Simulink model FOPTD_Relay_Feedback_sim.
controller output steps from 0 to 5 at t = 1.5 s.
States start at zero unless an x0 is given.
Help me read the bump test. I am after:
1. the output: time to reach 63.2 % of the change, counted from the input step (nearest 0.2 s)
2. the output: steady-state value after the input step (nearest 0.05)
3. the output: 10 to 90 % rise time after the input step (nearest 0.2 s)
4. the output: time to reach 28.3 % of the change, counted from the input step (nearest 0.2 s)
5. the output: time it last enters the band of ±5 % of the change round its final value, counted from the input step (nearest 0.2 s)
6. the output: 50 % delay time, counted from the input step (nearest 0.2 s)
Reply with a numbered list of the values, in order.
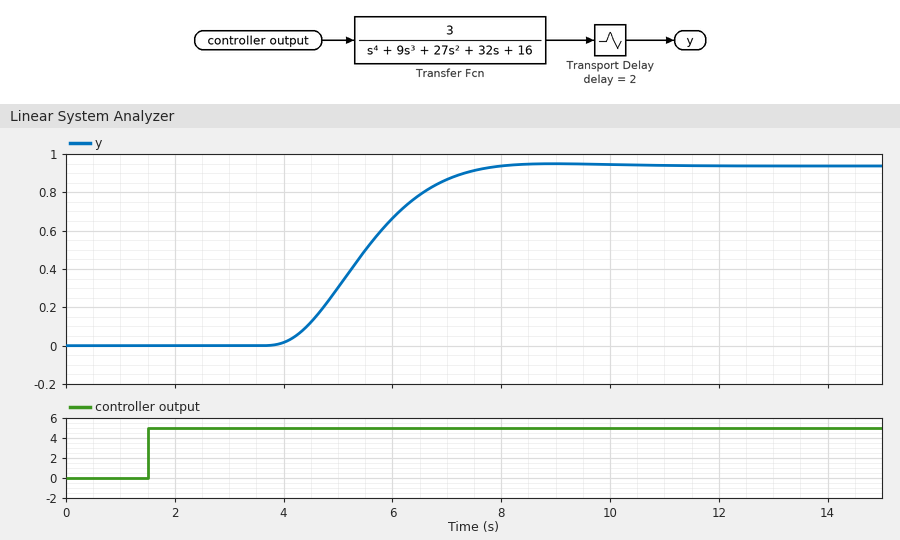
1. 4.2 s
2. 0.95
3. 2.4 s
4. 3.4 s
5. 5.8 s
6. 4.0 s
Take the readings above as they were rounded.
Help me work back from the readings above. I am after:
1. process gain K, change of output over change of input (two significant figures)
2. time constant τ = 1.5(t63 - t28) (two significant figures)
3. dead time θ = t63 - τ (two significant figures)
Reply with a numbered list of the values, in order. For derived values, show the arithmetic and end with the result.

1. (0.95 - 0) / 5 = 0.19
2. 1.5 × (4.2 - 3.4) = 1.2 s
3. 4.2 - 1.2 = 3.0 s
